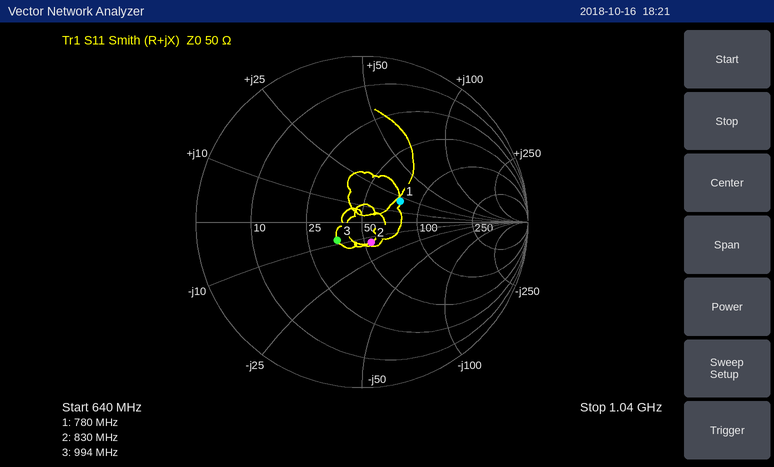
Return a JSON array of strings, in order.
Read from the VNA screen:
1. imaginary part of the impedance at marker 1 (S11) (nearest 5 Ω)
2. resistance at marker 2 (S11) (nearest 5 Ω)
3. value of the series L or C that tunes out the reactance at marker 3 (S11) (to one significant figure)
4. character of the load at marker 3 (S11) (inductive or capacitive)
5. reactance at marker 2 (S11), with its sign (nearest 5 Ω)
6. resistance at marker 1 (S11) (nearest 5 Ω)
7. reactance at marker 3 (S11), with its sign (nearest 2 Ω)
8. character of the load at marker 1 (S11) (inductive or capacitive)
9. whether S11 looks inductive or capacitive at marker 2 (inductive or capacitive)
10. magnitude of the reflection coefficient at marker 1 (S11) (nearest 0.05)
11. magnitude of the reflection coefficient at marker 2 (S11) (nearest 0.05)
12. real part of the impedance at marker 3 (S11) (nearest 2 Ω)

["+20 Ω", "55 Ω", "1 nH", "capacitive", "-15 Ω", "75 Ω", "-8 Ω", "inductive", "capacitive", "0.25", "0.15", "36 Ω"]
